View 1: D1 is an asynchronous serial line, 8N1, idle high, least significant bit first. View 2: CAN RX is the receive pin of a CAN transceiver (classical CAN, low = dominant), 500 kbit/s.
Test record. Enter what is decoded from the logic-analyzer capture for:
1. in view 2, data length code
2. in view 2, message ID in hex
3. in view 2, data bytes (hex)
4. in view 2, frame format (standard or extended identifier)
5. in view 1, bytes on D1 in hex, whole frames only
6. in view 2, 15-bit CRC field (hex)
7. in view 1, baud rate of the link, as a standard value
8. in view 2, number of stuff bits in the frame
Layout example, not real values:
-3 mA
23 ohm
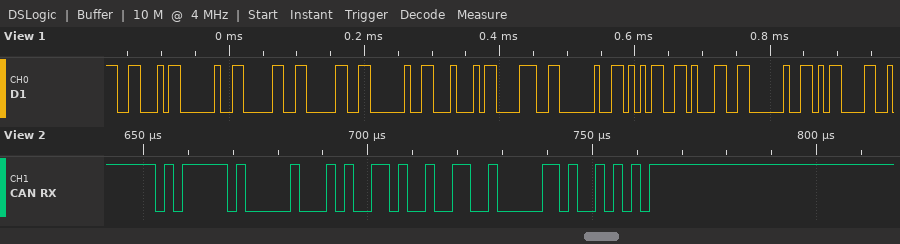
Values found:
2
0x5F8
9A 4C
standard
46 20 30 30 20 44 38 20 35 31 20 0D
0x414A
115200 baud
3
